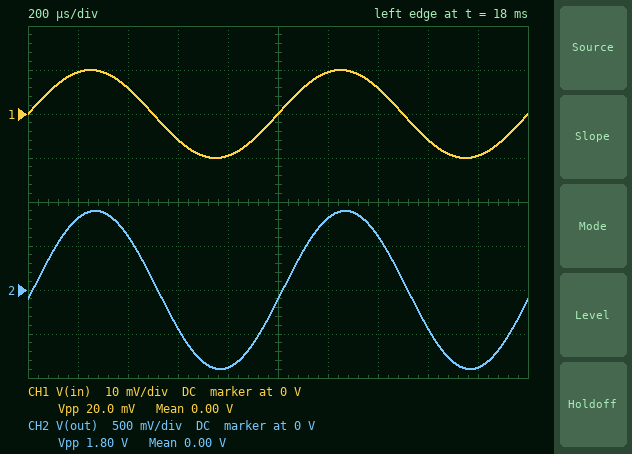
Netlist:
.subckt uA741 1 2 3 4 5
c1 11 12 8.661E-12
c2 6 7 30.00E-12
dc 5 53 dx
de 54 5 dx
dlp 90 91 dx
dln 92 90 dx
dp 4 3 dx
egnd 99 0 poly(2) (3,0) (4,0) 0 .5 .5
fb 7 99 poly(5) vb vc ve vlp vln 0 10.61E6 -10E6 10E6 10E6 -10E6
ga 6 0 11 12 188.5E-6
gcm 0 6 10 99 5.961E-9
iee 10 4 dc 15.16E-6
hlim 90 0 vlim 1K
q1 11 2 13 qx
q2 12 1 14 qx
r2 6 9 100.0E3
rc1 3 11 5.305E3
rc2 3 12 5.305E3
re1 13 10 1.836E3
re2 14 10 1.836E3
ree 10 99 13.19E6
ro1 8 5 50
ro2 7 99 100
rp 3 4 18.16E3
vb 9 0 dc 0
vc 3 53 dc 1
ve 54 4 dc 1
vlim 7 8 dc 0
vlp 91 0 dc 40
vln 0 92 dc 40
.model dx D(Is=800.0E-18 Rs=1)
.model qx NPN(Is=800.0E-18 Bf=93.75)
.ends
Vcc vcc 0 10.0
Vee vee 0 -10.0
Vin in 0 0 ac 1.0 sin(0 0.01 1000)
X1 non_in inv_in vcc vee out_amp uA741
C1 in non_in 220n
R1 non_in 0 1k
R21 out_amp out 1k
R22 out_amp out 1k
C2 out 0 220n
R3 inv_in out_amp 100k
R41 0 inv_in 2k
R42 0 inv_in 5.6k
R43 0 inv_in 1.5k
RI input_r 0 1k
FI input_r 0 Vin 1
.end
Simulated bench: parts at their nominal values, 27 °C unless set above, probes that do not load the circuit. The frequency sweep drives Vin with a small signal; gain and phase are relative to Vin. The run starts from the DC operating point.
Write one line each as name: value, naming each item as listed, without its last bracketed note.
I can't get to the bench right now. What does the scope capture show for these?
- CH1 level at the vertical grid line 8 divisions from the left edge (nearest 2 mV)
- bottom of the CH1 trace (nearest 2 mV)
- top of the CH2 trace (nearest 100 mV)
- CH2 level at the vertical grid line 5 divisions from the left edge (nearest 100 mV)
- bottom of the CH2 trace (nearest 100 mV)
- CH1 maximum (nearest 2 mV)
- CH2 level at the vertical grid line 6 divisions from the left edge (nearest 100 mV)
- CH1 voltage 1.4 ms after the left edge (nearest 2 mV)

CH1 level at the vertical grid line 8 divisions from the left edge: -6 mV
bottom of the CH1 trace: -10 mV
top of the CH2 trace: 900 mV
CH2 level at the vertical grid line 5 divisions from the left edge: -100 mV
bottom of the CH2 trace: -900 mV
CH1 maximum: 10 mV
CH2 level at the vertical grid line 6 divisions from the left edge: 800 mV
CH1 voltage 1.4 ms after the left edge: 6 mV
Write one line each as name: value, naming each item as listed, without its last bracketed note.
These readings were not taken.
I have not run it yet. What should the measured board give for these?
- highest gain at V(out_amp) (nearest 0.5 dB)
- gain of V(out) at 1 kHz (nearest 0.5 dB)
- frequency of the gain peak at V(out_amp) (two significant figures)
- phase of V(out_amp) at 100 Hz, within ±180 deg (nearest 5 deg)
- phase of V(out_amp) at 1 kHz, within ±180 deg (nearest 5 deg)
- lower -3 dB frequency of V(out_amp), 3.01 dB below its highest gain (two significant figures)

highest gain at V(out_amp): 42.0 dB
gain of V(out) at 1 kHz: 39.0 dB
frequency of the gain peak at V(out_amp): 2.2 kHz
phase of V(out_amp) at 100 Hz, within ±180 deg: 80 deg
phase of V(out_amp) at 1 kHz, within ±180 deg: 30 deg
lower -3 dB frequency of V(out_amp), 3.01 dB below its highest gain: 620 Hz
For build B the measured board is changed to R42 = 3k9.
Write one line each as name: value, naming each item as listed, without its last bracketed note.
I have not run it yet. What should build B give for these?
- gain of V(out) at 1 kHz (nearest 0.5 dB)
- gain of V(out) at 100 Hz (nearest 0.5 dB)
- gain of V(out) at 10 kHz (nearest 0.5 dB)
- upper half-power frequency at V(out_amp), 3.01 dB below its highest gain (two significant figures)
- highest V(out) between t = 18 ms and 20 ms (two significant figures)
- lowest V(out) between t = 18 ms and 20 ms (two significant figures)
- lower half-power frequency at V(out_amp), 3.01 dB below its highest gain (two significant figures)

gain of V(out) at 1 kHz: 39.5 dB
gain of V(out) at 100 Hz: 26.0 dB
gain of V(out) at 10 kHz: 21.0 dB
upper half-power frequency at V(out_amp), 3.01 dB below its highest gain: 7.6 kHz
highest V(out) between t = 18 ms and 20 ms: 950 mV
lowest V(out) between t = 18 ms and 20 ms: -950 mV
lower half-power frequency at V(out_amp), 3.01 dB below its highest gain: 610 Hz
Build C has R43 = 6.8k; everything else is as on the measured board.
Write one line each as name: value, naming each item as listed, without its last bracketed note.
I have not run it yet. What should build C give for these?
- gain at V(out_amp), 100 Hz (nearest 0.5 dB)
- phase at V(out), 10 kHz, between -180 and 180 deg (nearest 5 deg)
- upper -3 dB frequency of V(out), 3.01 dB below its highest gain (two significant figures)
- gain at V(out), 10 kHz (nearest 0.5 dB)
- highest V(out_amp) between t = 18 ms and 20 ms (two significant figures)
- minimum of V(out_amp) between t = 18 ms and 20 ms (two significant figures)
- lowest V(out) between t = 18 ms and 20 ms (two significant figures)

gain at V(out_amp), 100 Hz: 21.0 dB
phase at V(out), 10 kHz, between -180 and 180 deg: -120 deg
upper -3 dB frequency of V(out), 3.01 dB below its highest gain: 2.5 kHz
gain at V(out), 10 kHz: 19.0 dB
highest V(out_amp) between t = 18 ms and 20 ms: 680 mV
minimum of V(out_amp) between t = 18 ms and 20 ms: -670 mV
lowest V(out) between t = 18 ms and 20 ms: -550 mV
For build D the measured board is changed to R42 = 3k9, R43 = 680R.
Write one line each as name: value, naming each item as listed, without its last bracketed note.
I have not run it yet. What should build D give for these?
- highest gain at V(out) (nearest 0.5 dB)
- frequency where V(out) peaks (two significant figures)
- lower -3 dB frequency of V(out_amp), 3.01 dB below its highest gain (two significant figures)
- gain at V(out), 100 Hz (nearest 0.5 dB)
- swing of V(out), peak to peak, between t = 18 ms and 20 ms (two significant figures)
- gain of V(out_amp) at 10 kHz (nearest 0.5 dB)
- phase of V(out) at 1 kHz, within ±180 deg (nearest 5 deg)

highest gain at V(out): 43.5 dB
frequency where V(out) peaks: 980 Hz
lower -3 dB frequency of V(out_amp), 3.01 dB below its highest gain: 570 Hz
gain at V(out), 100 Hz: 29.5 dB
swing of V(out), peak to peak, between t = 18 ms and 20 ms: 2.9 V
gain of V(out_amp) at 10 kHz: 38.5 dB
phase of V(out) at 1 kHz, within ±180 deg: -10 deg
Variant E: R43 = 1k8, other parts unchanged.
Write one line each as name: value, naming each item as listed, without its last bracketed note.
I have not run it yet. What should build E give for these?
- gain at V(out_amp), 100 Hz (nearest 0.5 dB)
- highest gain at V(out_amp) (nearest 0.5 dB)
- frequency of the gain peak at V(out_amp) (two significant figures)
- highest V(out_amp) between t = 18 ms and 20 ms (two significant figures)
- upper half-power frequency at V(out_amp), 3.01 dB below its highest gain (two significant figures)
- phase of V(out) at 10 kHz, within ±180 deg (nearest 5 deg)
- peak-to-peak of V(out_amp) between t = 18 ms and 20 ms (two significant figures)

gain at V(out_amp), 100 Hz: 24.5 dB
highest gain at V(out_amp): 41.0 dB
frequency of the gain peak at V(out_amp): 2.3 kHz
highest V(out_amp) between t = 18 ms and 20 ms: 1.0 V
upper half-power frequency at V(out_amp), 3.01 dB below its highest gain: 8.6 kHz
phase of V(out) at 10 kHz, within ±180 deg: -130 deg
peak-to-peak of V(out_amp) between t = 18 ms and 20 ms: 2.0 V
